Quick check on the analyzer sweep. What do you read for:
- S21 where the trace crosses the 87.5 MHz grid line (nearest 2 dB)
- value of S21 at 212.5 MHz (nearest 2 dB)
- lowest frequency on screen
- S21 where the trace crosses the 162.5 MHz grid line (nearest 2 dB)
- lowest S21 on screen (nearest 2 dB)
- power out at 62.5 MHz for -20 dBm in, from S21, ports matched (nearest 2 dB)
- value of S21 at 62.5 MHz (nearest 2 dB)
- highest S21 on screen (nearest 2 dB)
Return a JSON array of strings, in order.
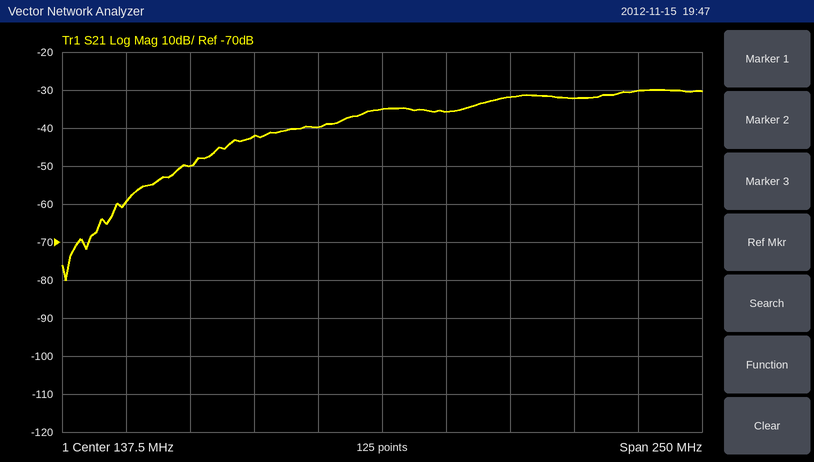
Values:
["-42 dB", "-32 dB", "12.5 MHz", "-36 dB", "-80 dB", "-70 dBm", "-50 dB", "-30 dB"]
